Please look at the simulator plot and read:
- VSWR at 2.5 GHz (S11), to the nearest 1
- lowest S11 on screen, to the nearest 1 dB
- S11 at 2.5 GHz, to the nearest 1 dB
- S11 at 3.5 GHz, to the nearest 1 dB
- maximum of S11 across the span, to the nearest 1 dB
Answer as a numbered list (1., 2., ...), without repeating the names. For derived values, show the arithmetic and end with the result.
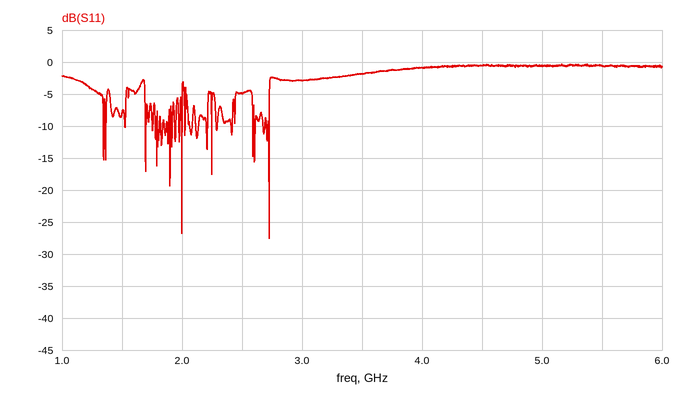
1. |Γ| = 10^(-5/20) = 0.5623; VSWR = (1 + 0.5623)/(1 − 0.5623) ≈ 4
2. -28 dB
3. -5 dB
4. -2 dB
5. 0 dB
